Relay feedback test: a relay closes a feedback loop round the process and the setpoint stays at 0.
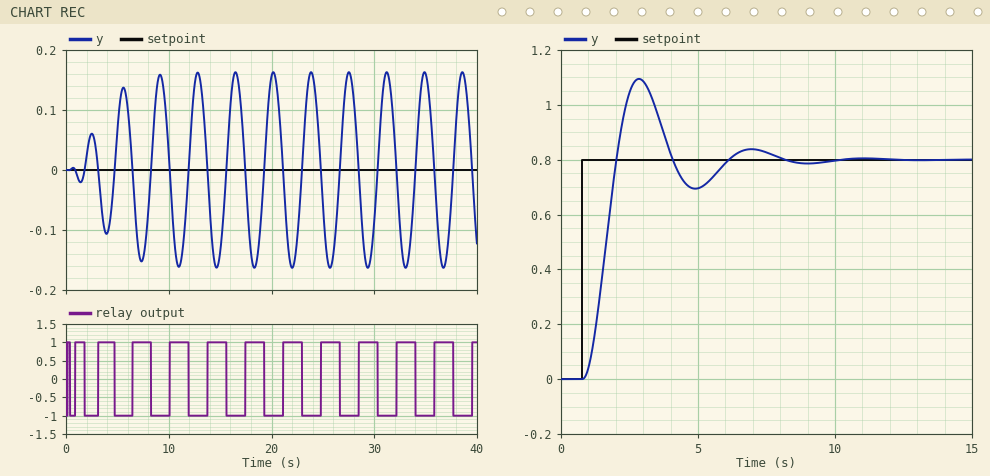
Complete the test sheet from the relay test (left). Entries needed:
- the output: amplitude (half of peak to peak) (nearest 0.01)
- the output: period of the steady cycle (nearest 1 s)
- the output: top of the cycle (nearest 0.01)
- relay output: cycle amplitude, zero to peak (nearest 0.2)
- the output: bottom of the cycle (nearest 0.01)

0.16
4 s
0.16
1.0
-0.16
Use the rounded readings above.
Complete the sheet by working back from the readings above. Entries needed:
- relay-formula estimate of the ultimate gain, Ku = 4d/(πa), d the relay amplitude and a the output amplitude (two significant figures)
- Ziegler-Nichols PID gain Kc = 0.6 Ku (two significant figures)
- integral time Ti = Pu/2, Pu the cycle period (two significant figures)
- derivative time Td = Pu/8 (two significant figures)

8.0
4.8
2.0 s
0.50 s
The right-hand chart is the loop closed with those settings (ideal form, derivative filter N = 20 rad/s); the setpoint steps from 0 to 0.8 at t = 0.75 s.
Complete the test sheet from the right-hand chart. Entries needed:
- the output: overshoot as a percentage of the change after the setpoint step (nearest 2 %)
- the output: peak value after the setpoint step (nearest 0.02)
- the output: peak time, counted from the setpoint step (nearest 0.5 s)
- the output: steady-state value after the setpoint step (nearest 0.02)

36 %
1.10
2.0 s
0.80
